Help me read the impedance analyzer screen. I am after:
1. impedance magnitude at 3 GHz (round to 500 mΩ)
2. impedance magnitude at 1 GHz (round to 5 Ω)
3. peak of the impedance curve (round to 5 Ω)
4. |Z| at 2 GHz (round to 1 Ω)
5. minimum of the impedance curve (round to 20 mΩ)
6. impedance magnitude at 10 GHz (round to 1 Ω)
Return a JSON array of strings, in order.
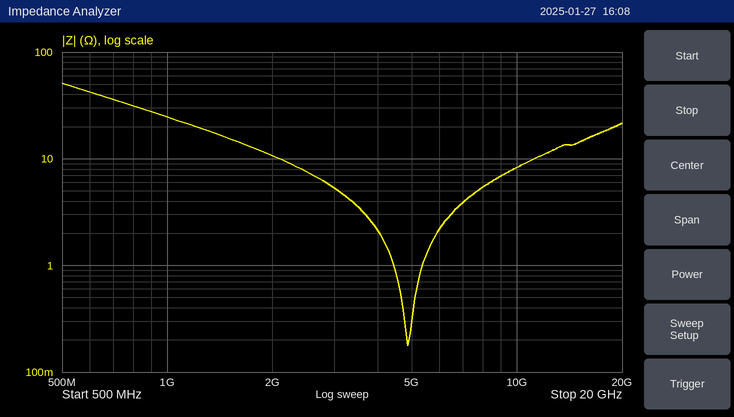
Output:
["5.5 Ω", "25 Ω", "50 Ω", "11 Ω", "180 mΩ", "8 Ω"]
